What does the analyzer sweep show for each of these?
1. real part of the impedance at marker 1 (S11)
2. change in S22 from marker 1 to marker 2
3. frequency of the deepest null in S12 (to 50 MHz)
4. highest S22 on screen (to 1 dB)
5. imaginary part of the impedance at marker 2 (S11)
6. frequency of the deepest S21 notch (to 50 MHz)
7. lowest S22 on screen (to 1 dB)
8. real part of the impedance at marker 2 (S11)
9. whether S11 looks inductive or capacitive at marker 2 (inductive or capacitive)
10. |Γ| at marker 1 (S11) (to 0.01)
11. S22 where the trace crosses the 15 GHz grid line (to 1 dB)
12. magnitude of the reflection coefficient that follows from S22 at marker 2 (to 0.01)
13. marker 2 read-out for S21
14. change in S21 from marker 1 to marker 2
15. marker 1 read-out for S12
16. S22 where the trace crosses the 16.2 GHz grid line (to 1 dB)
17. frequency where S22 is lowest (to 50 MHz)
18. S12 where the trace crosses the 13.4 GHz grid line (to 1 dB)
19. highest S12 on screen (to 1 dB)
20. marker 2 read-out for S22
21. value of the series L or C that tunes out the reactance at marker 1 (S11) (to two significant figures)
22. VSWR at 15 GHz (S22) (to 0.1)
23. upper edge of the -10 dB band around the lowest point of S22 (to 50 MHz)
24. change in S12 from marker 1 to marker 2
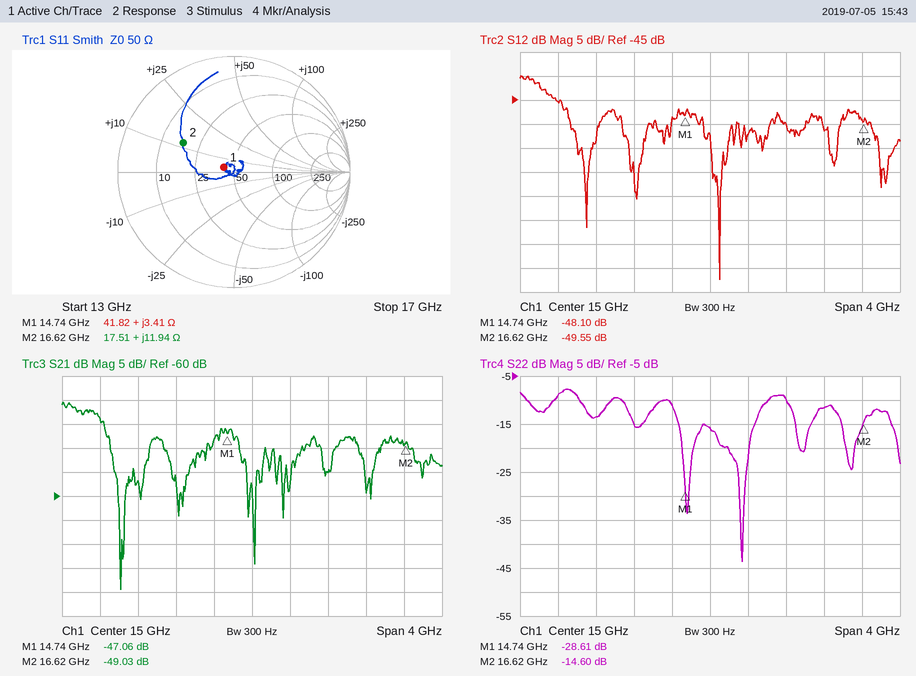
41.82 Ω
14.01 dB
15.10 GHz
-8 dB
+11.94 Ω
13.60 GHz
-44 dB
17.51 Ω
inductive
0.10
-16 dB
0.19
-49.03 dB
-1.97 dB
-48.10 dB
-12 dB
15.35 GHz
-45 dB
-40 dB
-14.60 dB
3.2 pF
1.4
15.60 GHz
-1.45 dB
